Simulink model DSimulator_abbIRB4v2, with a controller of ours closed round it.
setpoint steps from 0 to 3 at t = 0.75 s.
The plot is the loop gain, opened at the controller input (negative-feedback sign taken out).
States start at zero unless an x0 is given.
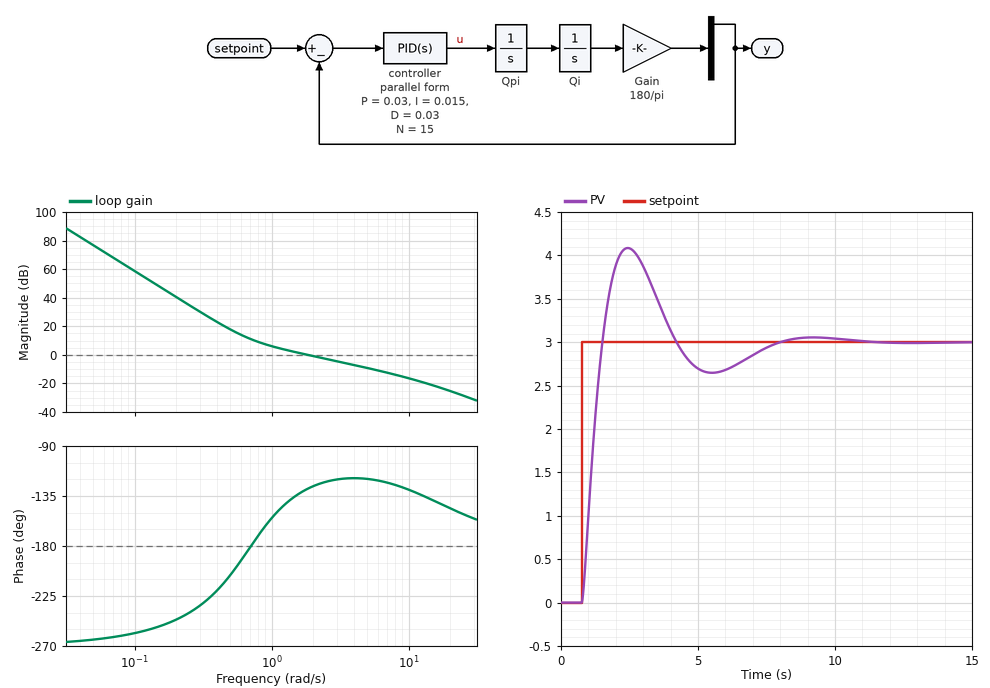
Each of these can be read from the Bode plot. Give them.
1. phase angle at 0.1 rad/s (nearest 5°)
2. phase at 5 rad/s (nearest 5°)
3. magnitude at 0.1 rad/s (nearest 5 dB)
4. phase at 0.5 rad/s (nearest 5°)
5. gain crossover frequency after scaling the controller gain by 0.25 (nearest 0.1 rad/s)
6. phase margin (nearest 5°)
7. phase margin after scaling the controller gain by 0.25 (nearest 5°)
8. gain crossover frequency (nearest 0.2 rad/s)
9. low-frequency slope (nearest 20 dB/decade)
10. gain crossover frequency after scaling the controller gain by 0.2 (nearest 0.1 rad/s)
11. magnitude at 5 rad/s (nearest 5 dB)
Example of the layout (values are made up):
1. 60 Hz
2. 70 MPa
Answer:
1. -260°
2. -120°
3. 60 dB
4. -205°
5. 0.7 rad/s
6. 50°
7. -5°
8. 1.8 rad/s
9. -60 dB/decade
10. 0.6 rad/s
11. -10 dB
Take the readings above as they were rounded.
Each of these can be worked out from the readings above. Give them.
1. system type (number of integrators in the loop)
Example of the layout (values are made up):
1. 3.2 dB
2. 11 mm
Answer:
1. 3
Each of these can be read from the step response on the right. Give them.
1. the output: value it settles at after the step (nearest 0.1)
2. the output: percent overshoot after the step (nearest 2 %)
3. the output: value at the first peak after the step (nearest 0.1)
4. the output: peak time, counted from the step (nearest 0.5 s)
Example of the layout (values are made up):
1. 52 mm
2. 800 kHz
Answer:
1. 3.0
2. 36 %
3. 4.1
4. 1.5 s
